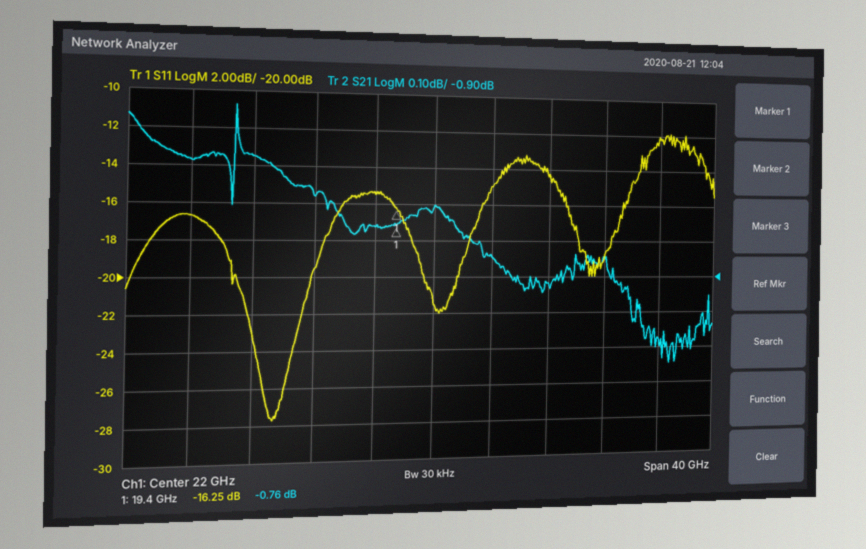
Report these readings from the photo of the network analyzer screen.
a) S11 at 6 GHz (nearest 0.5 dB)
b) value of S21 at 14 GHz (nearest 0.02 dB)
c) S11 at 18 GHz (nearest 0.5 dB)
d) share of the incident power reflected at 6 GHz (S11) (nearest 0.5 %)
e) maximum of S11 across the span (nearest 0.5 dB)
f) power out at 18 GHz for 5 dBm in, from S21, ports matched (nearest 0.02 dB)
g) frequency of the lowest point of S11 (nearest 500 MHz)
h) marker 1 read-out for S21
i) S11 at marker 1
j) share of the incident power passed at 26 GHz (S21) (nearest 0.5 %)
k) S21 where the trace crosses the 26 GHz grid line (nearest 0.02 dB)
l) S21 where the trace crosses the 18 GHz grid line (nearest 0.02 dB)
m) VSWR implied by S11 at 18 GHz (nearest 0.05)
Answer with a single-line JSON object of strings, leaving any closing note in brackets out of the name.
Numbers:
{"S11 at 6 GHz": "-16.5 dB", "value of S21 at 14 GHz": "-0.68 dB", "S11 at 18 GHz": "-15.5 dB", "share of the incident power reflected at 6 GHz (S11)": "2.0 %", "maximum of S11 across the span": "-12.0 dB", "power out at 18 GHz for 5 dBm in, from S21, ports matched": "4.24 dBm", "frequency of the lowest point of S11": "11.5 GHz", "marker 1 read-out for S21": "-0.76 dB", "S11 at marker 1": "-16.25 dB", "share of the incident power passed at 26 GHz (S21)": "82.5 %", "S21 where the trace crosses the 26 GHz grid line": "-0.84 dB", "S21 where the trace crosses the 18 GHz grid line": "-0.76 dB", "VSWR implied by S11 at 18 GHz": "1.40"}
